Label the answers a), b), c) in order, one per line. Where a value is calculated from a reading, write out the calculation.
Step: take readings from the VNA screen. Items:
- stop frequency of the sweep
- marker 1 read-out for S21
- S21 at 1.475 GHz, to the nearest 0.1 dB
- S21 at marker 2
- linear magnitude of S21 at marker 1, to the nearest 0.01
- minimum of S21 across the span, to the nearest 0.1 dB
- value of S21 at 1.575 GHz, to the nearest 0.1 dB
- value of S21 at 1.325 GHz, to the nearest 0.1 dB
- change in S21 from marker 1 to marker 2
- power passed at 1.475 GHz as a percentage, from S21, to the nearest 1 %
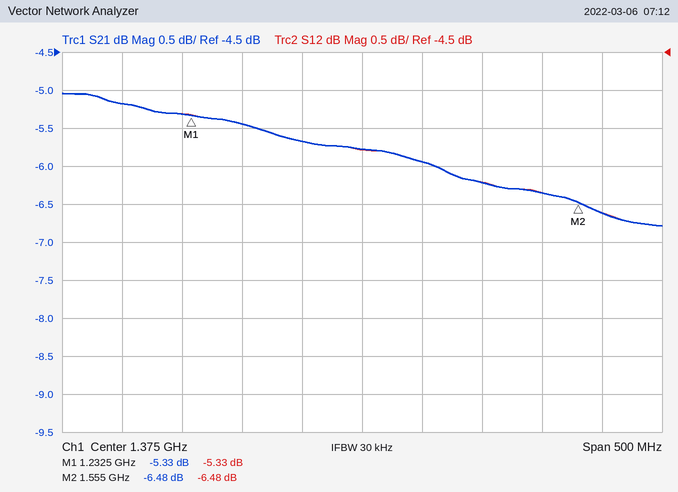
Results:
a) 1.625 GHz
b) -5.33 dB
c) -6.2 dB
d) -6.48 dB
e) 10^(-5.33/20) ≈ 0.54
f) -6.8 dB
g) -6.6 dB
h) -5.7 dB
i) -6.48 − (-5.33) = -1.15 dB
j) 10^(-6.2/10) ≈ 24 %
